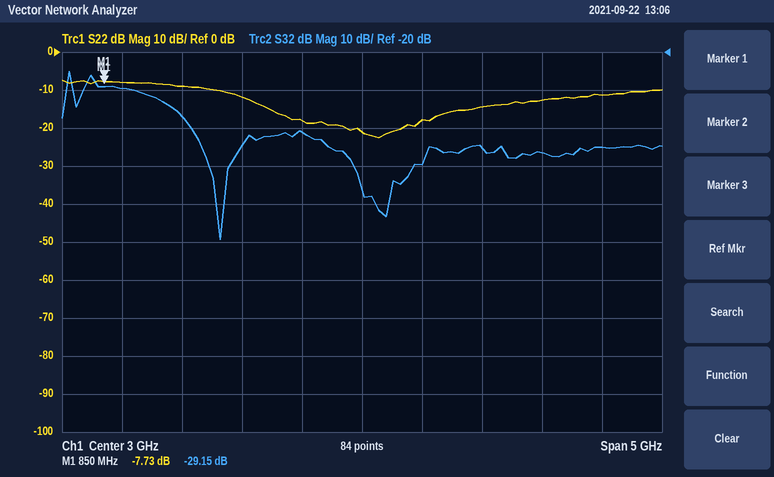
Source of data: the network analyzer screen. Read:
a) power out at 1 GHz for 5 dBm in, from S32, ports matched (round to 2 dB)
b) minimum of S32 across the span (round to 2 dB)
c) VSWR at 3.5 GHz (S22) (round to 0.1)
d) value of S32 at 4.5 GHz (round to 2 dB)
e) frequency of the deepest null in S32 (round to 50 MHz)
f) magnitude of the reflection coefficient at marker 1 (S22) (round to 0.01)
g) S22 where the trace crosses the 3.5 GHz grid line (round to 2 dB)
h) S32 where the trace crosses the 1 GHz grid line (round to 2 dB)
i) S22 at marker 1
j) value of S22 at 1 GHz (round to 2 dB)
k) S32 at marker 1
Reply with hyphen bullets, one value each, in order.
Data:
- -24 dBm
- -70 dB
- 1.3
- -46 dB
- 1.80 GHz
- 0.41
- -18 dB
- -30 dB
- -7.73 dB
- -8 dB
- -29.15 dB
